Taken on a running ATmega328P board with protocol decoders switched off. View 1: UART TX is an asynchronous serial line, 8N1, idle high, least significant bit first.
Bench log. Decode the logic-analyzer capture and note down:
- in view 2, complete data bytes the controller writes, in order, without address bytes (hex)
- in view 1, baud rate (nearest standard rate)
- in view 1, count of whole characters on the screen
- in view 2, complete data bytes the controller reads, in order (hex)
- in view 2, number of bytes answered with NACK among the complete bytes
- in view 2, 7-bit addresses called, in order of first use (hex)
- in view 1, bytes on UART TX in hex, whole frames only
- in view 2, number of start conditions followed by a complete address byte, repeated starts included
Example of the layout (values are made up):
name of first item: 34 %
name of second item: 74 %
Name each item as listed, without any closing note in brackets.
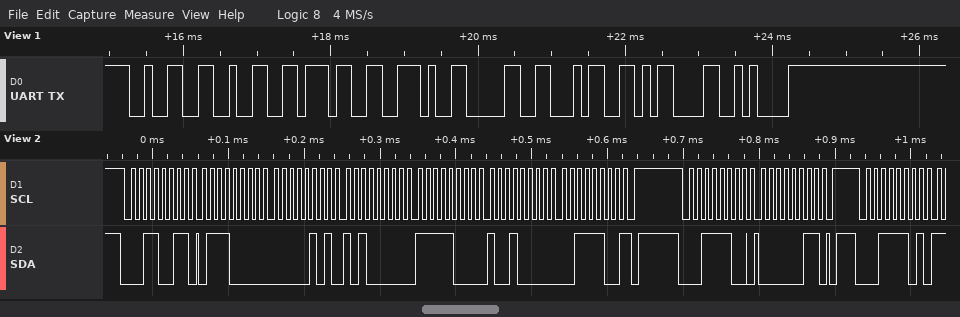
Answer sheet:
in view 2, complete data bytes the controller writes, in order, without address bytes: 03
in view 1, baud rate: 9600 baud
in view 1, count of whole characters on the screen: 8
in view 2, complete data bytes the controller reads, in order: 70 05 A0 F8 90 3C
in view 2, number of bytes answered with NACK among the complete bytes: 1
in view 2, 7-bit addresses called, in order of first use: 0x19 0x1E
in view 1, bytes on UART TX in hex, whole frames only: 0x32 0x32 0x37 0x2E 0x30 0x34 0x0D 0x0A
in view 2, number of start conditions followed by a complete address byte, repeated starts included: 3
